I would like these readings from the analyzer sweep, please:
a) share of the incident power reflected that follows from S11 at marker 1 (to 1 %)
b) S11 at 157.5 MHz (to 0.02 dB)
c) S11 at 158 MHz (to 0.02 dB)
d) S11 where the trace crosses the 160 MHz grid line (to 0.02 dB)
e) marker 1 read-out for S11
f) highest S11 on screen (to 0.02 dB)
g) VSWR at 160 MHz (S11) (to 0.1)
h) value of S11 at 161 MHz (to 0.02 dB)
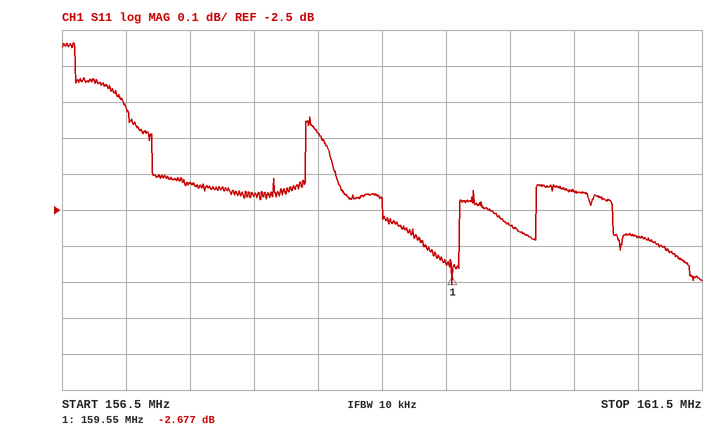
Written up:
54 %
-2.42 dB
-2.46 dB
-2.54 dB
-2.677 dB
-2.04 dB
6.9
-2.58 dB
